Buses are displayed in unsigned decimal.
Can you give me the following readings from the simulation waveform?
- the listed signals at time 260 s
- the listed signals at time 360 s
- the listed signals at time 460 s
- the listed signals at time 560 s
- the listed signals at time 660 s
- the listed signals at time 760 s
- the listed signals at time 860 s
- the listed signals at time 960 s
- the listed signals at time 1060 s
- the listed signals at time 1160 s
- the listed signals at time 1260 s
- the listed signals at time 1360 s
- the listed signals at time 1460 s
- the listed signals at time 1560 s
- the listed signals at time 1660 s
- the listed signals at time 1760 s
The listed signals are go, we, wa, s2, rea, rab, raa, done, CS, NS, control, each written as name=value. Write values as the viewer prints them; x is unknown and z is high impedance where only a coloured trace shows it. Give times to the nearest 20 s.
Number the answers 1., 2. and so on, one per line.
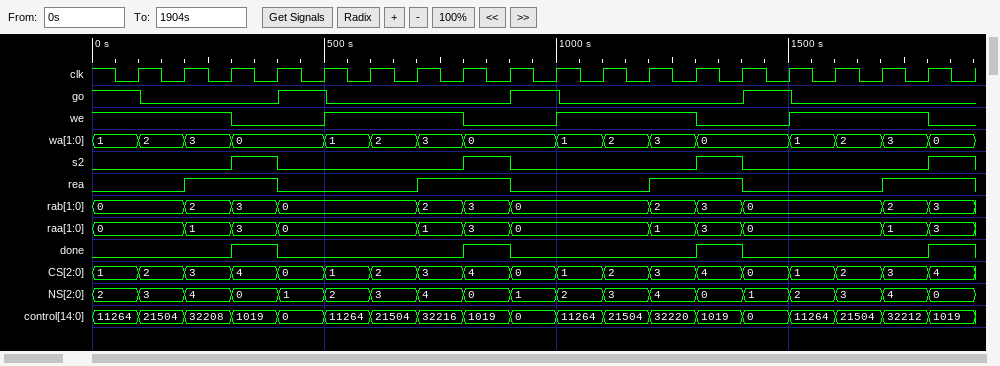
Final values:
1. go=0, we=1, wa=3, s2=0, rea=1, rab=2, raa=1, done=0, CS=3, NS=4, control=32208
2. go=0, we=0, wa=0, s2=1, rea=1, rab=3, raa=3, done=1, CS=4, NS=0, control=1019
3. go=1, we=0, wa=0, s2=0, rea=0, rab=0, raa=0, done=0, CS=0, NS=1, control=0
4. go=0, we=1, wa=1, s2=0, rea=0, rab=0, raa=0, done=0, CS=1, NS=2, control=11264
5. go=0, we=1, wa=2, s2=0, rea=0, rab=0, raa=0, done=0, CS=2, NS=3, control=21504
6. go=0, we=1, wa=3, s2=0, rea=1, rab=2, raa=1, done=0, CS=3, NS=4, control=32216
7. go=0, we=0, wa=0, s2=1, rea=1, rab=3, raa=3, done=1, CS=4, NS=0, control=1019
8. go=1, we=0, wa=0, s2=0, rea=0, rab=0, raa=0, done=0, CS=0, NS=1, control=0
9. go=0, we=1, wa=1, s2=0, rea=0, rab=0, raa=0, done=0, CS=1, NS=2, control=11264
10. go=0, we=1, wa=2, s2=0, rea=0, rab=0, raa=0, done=0, CS=2, NS=3, control=21504
11. go=0, we=1, wa=3, s2=0, rea=1, rab=2, raa=1, done=0, CS=3, NS=4, control=32220
12. go=0, we=0, wa=0, s2=1, rea=1, rab=3, raa=3, done=1, CS=4, NS=0, control=1019
13. go=1, we=0, wa=0, s2=0, rea=0, rab=0, raa=0, done=0, CS=0, NS=1, control=0
14. go=0, we=1, wa=1, s2=0, rea=0, rab=0, raa=0, done=0, CS=1, NS=2, control=11264
15. go=0, we=1, wa=2, s2=0, rea=0, rab=0, raa=0, done=0, CS=2, NS=3, control=21504
16. go=0, we=1, wa=3, s2=0, rea=1, rab=2, raa=1, done=0, CS=3, NS=4, control=32212
